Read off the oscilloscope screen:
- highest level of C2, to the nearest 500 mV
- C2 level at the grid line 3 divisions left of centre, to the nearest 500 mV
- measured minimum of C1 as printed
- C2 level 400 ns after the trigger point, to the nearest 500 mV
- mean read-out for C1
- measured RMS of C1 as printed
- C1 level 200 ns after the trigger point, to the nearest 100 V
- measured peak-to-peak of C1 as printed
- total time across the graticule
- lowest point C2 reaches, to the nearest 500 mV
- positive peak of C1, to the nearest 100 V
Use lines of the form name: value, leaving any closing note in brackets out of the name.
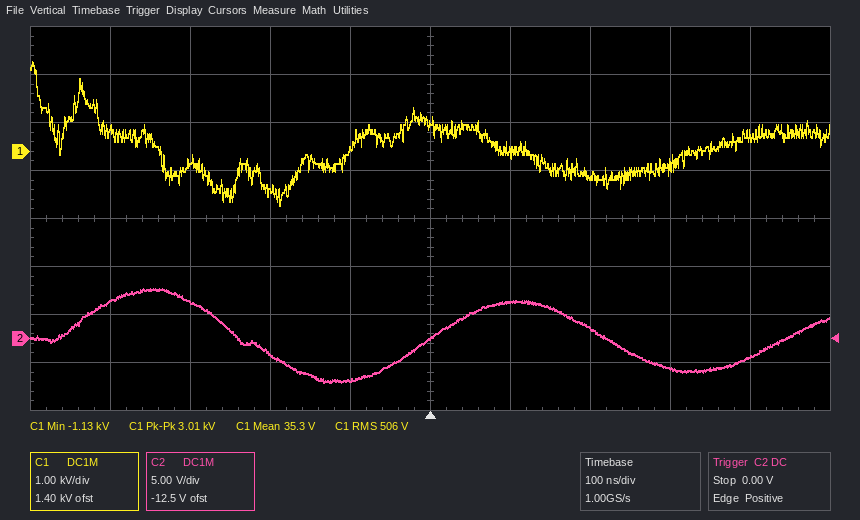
highest level of C2, to the nearest 500 mV: 5.0 V
C2 level at the grid line 3 divisions left of centre, to the nearest 500 mV: 4.0 V
measured minimum of C1 as printed: -1.13 kV
C2 level 400 ns after the trigger point, to the nearest 500 mV: -2.0 V
mean read-out for C1: 35.3 V
measured RMS of C1 as printed: 506 V
C1 level 200 ns after the trigger point, to the nearest 100 V: -500 V
measured peak-to-peak of C1 as printed: 3.01 kV
total time across the graticule: 1 µs
lowest point C2 reaches, to the nearest 500 mV: -4.5 V
positive peak of C1, to the nearest 100 V: 1.9 kV
